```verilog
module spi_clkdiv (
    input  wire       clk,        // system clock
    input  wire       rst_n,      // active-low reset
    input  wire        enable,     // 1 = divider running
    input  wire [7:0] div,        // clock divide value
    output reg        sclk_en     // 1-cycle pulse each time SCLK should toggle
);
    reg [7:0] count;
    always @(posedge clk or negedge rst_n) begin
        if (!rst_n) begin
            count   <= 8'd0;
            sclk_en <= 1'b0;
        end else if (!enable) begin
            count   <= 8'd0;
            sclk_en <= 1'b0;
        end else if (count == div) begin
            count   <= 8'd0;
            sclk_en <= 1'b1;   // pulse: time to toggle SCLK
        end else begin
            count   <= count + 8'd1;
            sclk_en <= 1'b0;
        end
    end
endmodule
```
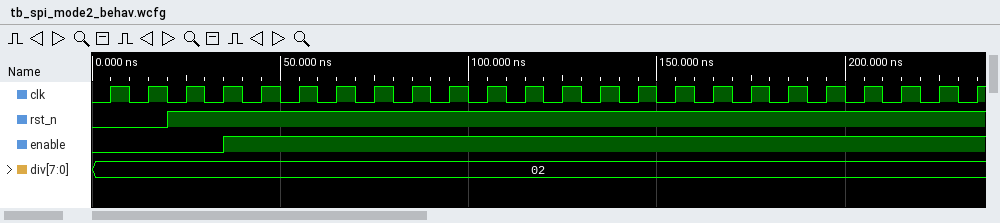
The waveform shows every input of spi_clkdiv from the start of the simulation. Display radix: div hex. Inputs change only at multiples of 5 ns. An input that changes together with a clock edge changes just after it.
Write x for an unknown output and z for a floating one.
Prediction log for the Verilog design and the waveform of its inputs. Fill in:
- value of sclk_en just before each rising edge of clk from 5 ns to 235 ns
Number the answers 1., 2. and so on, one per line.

1. 0 0 0 0 0 0 0 1 0 0 1 0 0 1 0 0 1 0 0 1 0 0 1 0
